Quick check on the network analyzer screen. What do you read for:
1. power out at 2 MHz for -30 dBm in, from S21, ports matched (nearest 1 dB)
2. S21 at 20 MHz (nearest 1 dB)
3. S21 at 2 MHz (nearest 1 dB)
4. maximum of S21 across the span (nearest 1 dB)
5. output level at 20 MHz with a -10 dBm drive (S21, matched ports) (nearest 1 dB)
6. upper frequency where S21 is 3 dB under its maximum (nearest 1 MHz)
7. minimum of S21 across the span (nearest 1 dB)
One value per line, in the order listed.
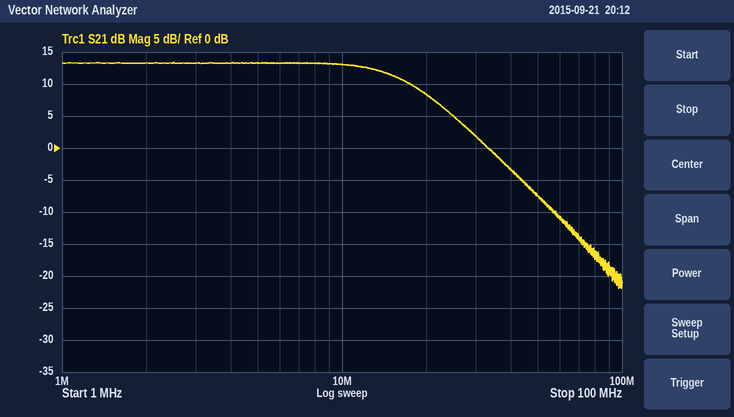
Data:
-17 dBm
8 dB
13 dB
13 dB
-2 dBm
17 MHz
-22 dB
